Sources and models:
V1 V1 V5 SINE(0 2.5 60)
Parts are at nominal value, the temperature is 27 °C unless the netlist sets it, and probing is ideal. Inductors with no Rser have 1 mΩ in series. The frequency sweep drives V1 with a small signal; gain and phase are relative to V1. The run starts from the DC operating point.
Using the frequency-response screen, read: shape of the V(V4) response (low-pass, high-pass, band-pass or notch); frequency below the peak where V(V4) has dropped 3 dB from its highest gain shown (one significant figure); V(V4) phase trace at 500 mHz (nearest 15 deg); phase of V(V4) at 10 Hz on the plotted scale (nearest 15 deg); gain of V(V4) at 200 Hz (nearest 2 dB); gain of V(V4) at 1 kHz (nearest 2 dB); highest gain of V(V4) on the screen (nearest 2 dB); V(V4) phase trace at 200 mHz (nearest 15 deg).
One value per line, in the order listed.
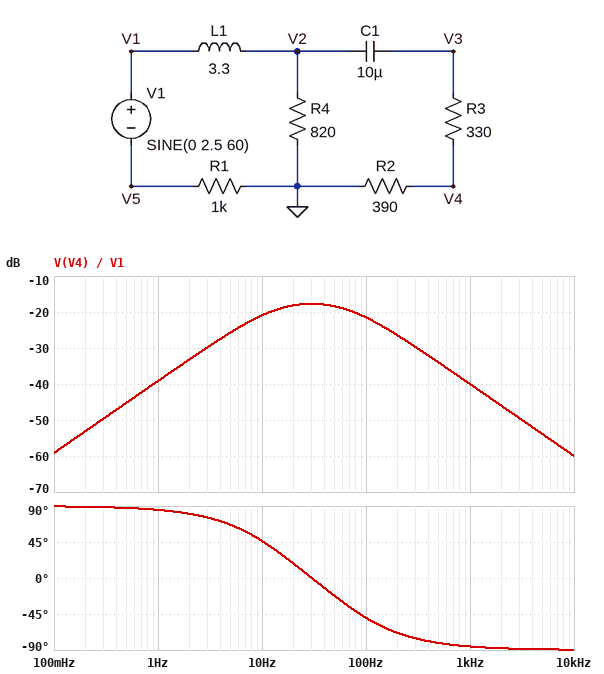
band-pass
10 Hz
90 deg
45 deg
-26 dB
-40 dB
-18 dB
90 deg
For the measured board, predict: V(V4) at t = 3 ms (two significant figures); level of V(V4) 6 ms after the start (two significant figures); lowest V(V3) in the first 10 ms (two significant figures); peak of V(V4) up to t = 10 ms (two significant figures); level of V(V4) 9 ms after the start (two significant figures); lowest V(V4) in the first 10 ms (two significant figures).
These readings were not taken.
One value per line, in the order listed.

150 mV
230 mV
-130 mV
240 mV
32 mV
-71 mV
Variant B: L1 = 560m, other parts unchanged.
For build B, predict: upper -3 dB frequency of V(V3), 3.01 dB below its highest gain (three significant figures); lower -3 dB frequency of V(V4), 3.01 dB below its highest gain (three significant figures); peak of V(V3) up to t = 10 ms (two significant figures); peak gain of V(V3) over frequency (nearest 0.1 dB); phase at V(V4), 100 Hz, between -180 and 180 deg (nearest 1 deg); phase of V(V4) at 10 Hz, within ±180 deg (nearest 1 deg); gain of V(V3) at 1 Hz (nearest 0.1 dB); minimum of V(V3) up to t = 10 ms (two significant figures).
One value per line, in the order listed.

416 Hz
12.8 Hz
560 mV
-11.4 dB
-7 deg
52 deg
-33.8 dB
-500 mV
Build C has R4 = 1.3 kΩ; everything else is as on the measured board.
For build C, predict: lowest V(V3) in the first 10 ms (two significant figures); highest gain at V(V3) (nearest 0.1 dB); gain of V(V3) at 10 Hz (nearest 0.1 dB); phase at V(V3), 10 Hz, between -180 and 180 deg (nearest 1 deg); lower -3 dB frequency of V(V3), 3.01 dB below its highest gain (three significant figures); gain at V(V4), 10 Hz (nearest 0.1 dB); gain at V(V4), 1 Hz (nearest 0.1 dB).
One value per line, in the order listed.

-150 mV
-10.9 dB
-13.9 dB
45 deg
9.89 Hz
-19.2 dB
-37.2 dB
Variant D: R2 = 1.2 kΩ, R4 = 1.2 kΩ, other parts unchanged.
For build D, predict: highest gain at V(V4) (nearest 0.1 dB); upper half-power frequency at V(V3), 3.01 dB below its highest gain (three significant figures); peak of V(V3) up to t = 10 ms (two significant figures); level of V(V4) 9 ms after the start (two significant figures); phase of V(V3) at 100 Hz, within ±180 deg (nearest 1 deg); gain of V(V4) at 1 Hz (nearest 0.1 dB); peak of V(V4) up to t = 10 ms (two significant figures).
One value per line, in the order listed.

-10.6 dB
93.1 Hz
740 mV
100 mV
-47 deg
-27.8 dB
580 mV
